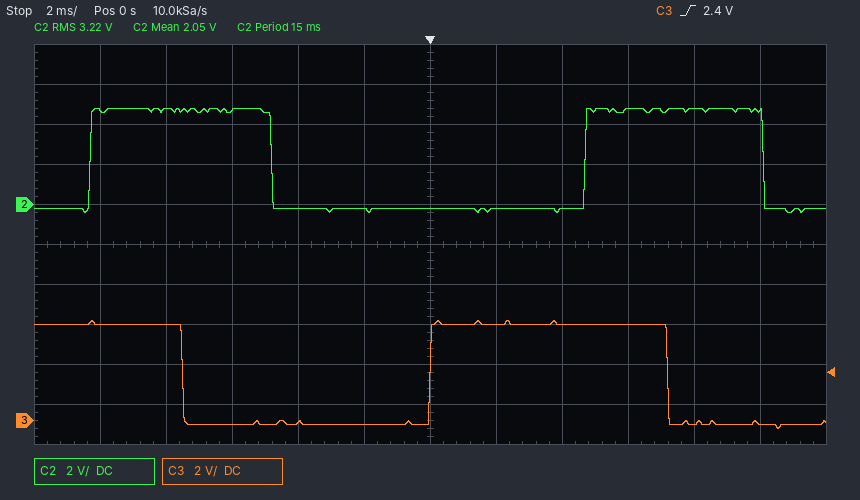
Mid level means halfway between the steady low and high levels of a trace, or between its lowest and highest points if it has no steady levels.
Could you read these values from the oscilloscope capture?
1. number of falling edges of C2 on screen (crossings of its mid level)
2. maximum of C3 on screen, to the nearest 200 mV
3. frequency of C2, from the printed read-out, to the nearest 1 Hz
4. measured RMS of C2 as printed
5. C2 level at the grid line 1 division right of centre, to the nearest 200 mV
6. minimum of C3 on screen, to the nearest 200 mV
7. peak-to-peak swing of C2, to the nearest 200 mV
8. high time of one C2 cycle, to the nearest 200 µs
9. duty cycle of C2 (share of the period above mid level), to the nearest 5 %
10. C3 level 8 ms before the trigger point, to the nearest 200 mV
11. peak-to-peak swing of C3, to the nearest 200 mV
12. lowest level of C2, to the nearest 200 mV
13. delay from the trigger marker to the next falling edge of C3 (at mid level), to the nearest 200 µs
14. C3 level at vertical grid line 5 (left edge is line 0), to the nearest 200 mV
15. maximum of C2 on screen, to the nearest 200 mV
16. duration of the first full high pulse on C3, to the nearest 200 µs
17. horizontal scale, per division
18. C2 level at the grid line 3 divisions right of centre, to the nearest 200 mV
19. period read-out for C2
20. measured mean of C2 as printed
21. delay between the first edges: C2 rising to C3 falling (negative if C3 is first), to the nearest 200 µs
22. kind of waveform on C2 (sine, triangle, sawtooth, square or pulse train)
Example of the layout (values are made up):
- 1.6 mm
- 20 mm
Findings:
- 2
- 5.0 V
- 67 Hz
- 3.22 V
- -200 mV
- -400 mV
- 5.2 V
- 5.4 ms
- 35 %
- 4.8 V
- 5.4 V
- -400 mV
- 7.2 ms
- -200 mV
- 4.8 V
- 7.2 ms
- 2 ms
- 4.8 V
- 15 ms
- 2.05 V
- +2.8 ms
- pulse train
